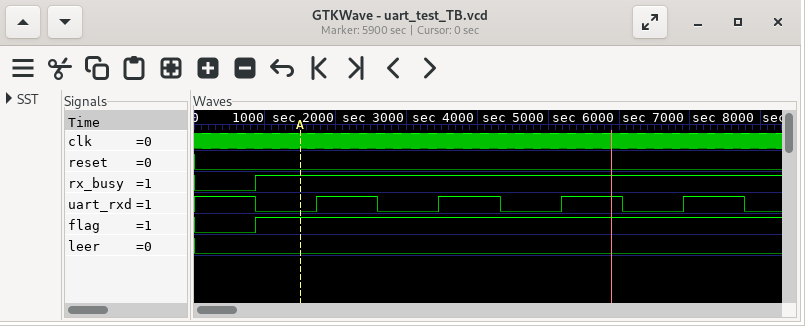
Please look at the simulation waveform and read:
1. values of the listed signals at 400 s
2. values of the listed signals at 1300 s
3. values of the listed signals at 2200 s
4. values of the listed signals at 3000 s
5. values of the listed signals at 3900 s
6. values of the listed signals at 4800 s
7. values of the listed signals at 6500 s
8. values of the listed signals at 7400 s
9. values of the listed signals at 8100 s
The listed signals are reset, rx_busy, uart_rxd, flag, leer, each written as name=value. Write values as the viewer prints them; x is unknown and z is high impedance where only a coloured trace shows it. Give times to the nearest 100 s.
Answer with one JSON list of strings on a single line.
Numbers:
["reset=0, rx_busy=0, uart_rxd=1, flag=0, leer=0", "reset=0, rx_busy=1, uart_rxd=0, flag=1, leer=0", "reset=0, rx_busy=1, uart_rxd=1, flag=1, leer=0", "reset=0, rx_busy=1, uart_rxd=0, flag=1, leer=0", "reset=0, rx_busy=1, uart_rxd=1, flag=1, leer=0", "reset=0, rx_busy=1, uart_rxd=0, flag=1, leer=0", "reset=0, rx_busy=1, uart_rxd=0, flag=1, leer=0", "reset=0, rx_busy=1, uart_rxd=1, flag=1, leer=0", "reset=0, rx_busy=1, uart_rxd=0, flag=1, leer=0"]
